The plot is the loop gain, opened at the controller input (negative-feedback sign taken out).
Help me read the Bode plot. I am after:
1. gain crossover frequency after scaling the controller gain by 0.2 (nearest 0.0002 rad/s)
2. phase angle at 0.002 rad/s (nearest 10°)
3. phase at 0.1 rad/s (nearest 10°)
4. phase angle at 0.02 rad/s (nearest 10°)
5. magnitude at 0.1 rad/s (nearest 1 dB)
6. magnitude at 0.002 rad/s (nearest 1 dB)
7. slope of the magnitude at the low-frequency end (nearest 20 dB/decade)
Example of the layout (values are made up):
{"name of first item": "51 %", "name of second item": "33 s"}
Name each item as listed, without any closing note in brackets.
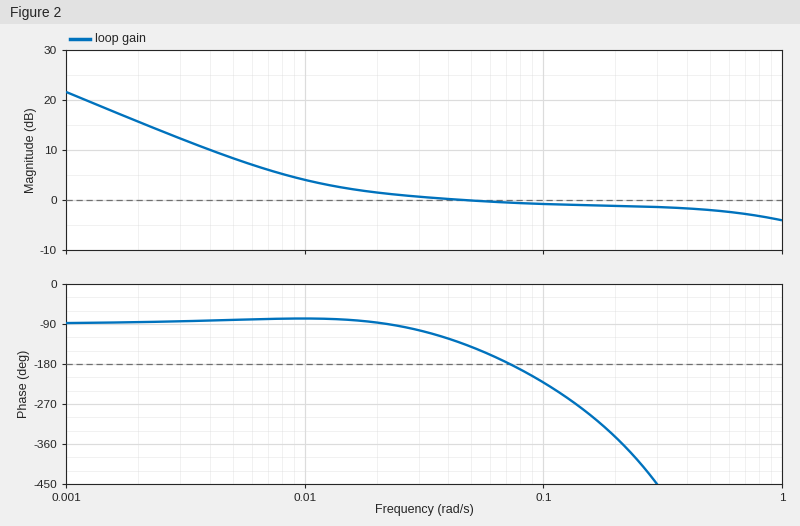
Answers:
{"gain crossover frequency after scaling the controller gain by 0.2": "0.0024 rad/s", "phase angle at 0.002 rad/s": "-90°", "phase at 0.1 rad/s": "-220°", "phase angle at 0.02 rad/s": "-90°", "magnitude at 0.1 rad/s": "-1 dB", "magnitude at 0.002 rad/s": "16 dB", "slope of the magnitude at the low-frequency end": "-20 dB/decade"}
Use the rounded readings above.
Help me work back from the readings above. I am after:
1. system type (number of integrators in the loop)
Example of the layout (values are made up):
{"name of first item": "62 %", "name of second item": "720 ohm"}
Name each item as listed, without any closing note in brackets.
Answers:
{"system type": "1"}
